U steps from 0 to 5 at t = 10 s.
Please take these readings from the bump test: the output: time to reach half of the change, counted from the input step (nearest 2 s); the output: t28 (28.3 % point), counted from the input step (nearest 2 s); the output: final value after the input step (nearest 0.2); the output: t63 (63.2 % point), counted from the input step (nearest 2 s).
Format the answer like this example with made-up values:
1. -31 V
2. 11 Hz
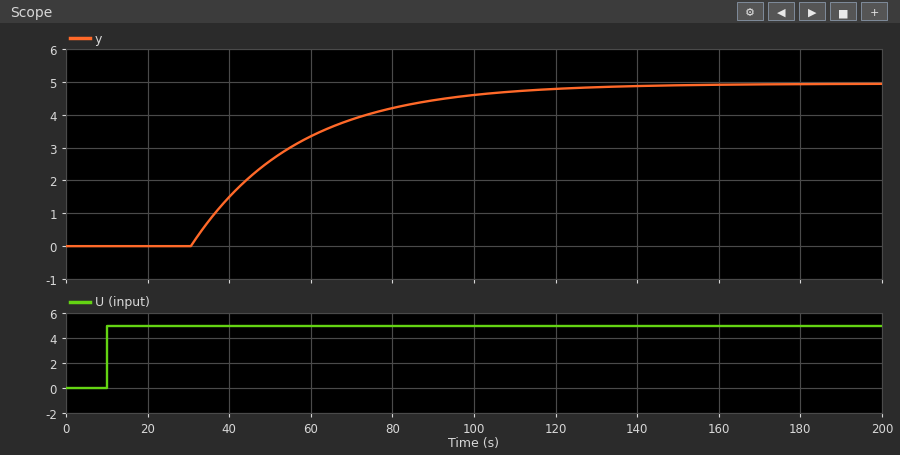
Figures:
1. 38 s
2. 30 s
3. 5.0
4. 46 s
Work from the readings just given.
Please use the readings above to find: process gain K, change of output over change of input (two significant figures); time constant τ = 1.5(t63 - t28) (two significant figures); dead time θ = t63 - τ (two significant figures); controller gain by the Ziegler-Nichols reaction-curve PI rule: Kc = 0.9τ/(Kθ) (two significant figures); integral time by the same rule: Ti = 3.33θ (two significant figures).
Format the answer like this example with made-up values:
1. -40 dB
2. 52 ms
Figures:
1. 1.0
2. 24 s
3. 22 s
4. 0.98
5. 73 s
